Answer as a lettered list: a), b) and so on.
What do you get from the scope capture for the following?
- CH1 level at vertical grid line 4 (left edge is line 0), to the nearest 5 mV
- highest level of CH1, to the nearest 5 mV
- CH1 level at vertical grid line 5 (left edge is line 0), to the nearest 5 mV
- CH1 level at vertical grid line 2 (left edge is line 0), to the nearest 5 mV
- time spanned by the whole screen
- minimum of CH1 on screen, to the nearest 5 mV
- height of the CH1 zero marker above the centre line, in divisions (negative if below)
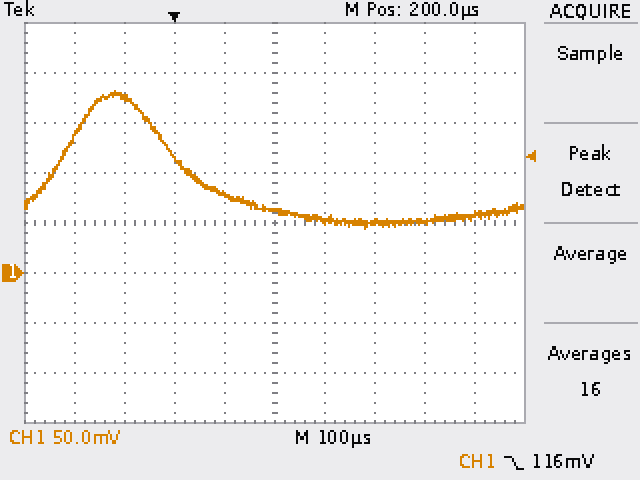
a) 80 mV
b) 180 mV
c) 65 mV
d) 175 mV
e) 1 ms
f) 45 mV
g) -1.0 div
